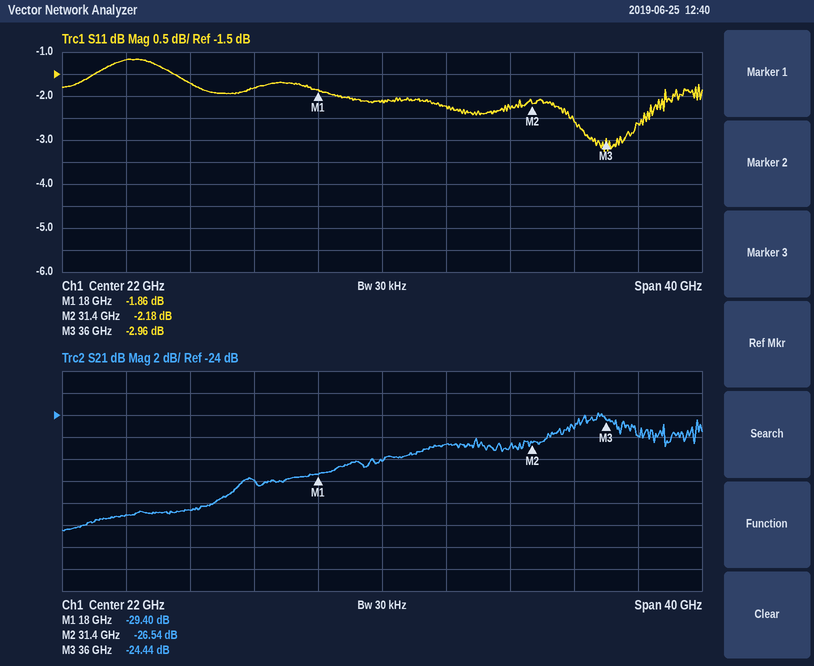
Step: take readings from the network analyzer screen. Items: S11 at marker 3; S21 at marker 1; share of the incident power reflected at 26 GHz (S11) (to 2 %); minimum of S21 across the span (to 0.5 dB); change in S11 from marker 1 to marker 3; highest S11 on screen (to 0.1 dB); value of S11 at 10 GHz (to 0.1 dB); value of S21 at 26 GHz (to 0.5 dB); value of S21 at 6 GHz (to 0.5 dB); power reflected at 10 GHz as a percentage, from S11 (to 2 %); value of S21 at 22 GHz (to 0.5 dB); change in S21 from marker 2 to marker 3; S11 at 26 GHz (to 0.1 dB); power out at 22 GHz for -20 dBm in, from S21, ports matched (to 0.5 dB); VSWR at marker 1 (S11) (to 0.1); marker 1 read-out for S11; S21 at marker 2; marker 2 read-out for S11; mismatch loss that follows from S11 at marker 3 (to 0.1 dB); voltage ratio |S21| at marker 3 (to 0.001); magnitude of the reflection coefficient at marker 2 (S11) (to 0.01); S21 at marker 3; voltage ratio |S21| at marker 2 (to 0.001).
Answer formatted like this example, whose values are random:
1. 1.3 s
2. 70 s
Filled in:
1. -2.96 dB
2. -29.40 dB
3. 60 %
4. -34.5 dB
5. -1.10 dB
6. -1.2 dB
7. -1.7 dB
8. -26.5 dB
9. -33.0 dB
10. 68 %
11. -28.0 dB
12. 2.10 dB
13. -2.2 dB
14. -48.0 dBm
15. 9.4
16. -1.86 dB
17. -26.54 dB
18. -2.18 dB
19. 3.1 dB
20. 0.060
21. 0.78
22. -24.44 dB
23. 0.047
